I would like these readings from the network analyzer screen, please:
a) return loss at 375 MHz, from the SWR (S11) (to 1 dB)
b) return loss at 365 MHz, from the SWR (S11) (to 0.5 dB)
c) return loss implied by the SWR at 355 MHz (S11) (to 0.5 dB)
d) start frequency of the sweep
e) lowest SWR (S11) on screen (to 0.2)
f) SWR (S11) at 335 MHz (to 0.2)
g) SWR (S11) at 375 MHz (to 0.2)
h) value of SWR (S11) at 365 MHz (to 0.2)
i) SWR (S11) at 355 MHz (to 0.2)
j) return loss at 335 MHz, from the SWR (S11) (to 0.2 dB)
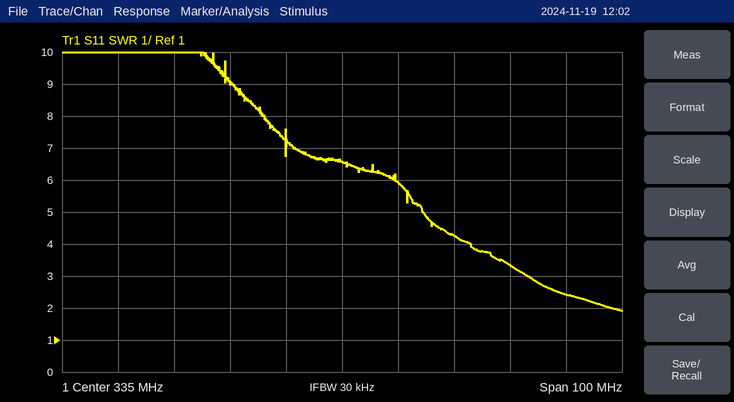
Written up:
8 dB
5.5 dB
4.0 dB
285 MHz
2.0
6.6
2.4
3.4
4.2
2.6 dB
